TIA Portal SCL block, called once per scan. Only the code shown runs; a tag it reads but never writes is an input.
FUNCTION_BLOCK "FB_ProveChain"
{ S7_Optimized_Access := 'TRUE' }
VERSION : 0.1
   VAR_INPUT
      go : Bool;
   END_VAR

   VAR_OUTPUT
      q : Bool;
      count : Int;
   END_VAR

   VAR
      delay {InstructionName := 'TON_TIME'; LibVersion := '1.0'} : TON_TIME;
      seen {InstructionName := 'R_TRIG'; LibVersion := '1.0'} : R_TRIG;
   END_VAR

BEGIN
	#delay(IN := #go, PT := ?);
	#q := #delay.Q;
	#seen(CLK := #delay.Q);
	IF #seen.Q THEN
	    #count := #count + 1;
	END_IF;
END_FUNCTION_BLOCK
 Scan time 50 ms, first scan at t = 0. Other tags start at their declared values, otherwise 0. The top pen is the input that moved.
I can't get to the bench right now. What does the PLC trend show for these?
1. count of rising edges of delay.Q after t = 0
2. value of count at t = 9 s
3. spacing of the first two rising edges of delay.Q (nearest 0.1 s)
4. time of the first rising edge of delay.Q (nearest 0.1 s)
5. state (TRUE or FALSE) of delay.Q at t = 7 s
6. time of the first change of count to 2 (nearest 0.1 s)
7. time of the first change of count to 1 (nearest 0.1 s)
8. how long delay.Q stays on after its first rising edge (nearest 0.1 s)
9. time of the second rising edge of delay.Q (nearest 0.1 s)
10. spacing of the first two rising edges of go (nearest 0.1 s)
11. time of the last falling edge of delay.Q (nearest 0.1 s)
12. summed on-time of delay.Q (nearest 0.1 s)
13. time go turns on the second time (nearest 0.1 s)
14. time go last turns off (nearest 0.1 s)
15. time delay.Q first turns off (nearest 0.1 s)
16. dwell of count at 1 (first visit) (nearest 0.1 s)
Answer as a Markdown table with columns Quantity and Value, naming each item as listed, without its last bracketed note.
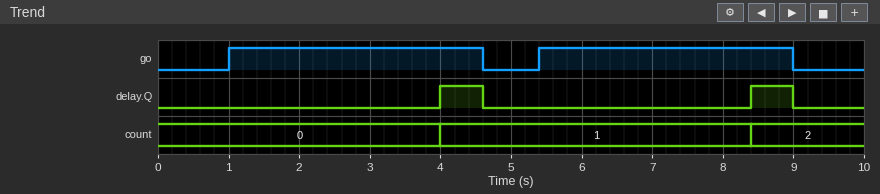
| Quantity | Value |
|---|---|
| count of rising edges of delay.Q after t = 0 | 2 |
| value of count at t = 9 s | 2 |
| spacing of the first two rising edges of delay.Q | 4.4 s |
| time of the first rising edge of delay.Q | 4.0 s |
| state (TRUE or FALSE) of delay.Q at t = 7 s | FALSE |
| time of the first change of count to 2 | 8.4 s |
| time of the first change of count to 1 | 4.0 s |
| how long delay.Q stays on after its first rising edge | 0.6 s |
| time of the second rising edge of delay.Q | 8.4 s |
| spacing of the first two rising edges of go | 4.4 s |
| time of the last falling edge of delay.Q | 9.0 s |
| summed on-time of delay.Q | 1.2 s |
| time go turns on the second time | 5.4 s |
| time go last turns off | 9.0 s |
| time delay.Q first turns off | 4.6 s |
| dwell of count at 1 (first visit) | 4.4 s |
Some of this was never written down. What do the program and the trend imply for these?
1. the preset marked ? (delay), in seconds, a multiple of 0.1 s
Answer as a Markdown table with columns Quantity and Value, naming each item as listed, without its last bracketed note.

| Quantity | Value |
|---|---|
| the preset marked ? (delay), in seconds, a multiple of 0.1 s | 3.0 s |
